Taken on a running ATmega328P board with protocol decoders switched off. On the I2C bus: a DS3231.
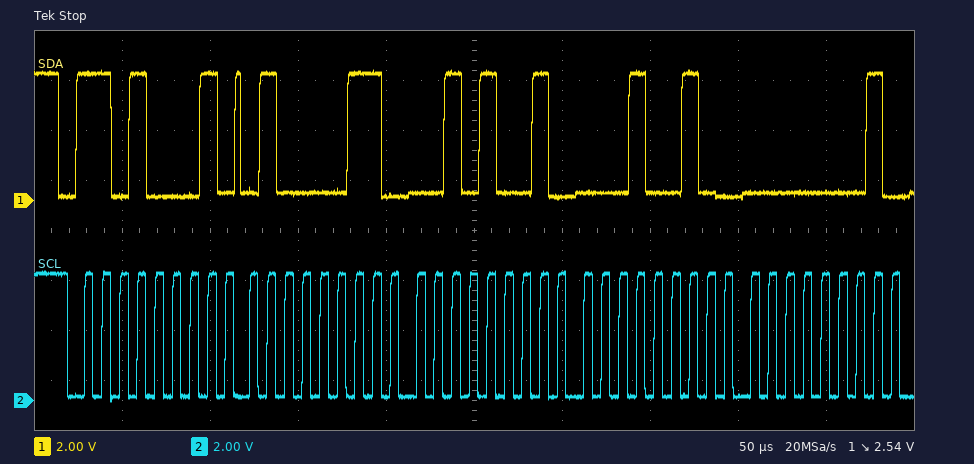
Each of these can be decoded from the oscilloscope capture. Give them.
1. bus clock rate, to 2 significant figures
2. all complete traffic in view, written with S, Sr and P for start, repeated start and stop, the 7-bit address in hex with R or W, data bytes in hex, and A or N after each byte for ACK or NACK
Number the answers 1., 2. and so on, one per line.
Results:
1. 100 kHz
2. S 68R A 43 A 29 A 12 A 01 A
